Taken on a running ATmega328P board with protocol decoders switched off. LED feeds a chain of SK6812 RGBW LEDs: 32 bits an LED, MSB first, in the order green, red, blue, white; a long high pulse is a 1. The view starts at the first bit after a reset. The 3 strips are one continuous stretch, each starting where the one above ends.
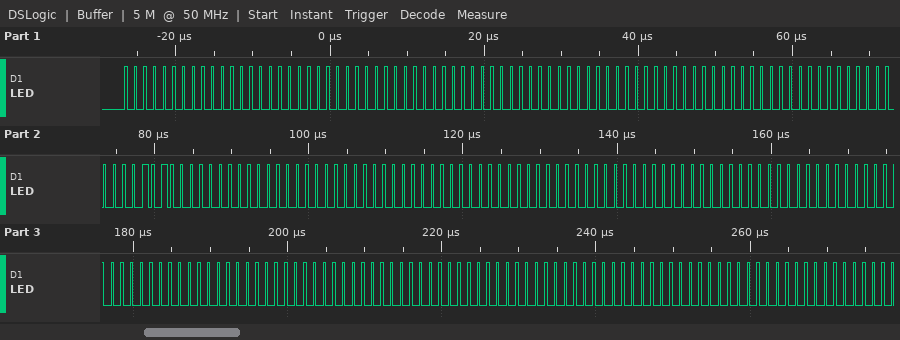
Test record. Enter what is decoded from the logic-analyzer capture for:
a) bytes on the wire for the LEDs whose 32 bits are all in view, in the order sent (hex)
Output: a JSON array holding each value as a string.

["00 00 00 00 00 00 00 00 00 00 0A 00 00 00 00 00 00 00 00 00 00 00 00 00 00 00 00 00"]
